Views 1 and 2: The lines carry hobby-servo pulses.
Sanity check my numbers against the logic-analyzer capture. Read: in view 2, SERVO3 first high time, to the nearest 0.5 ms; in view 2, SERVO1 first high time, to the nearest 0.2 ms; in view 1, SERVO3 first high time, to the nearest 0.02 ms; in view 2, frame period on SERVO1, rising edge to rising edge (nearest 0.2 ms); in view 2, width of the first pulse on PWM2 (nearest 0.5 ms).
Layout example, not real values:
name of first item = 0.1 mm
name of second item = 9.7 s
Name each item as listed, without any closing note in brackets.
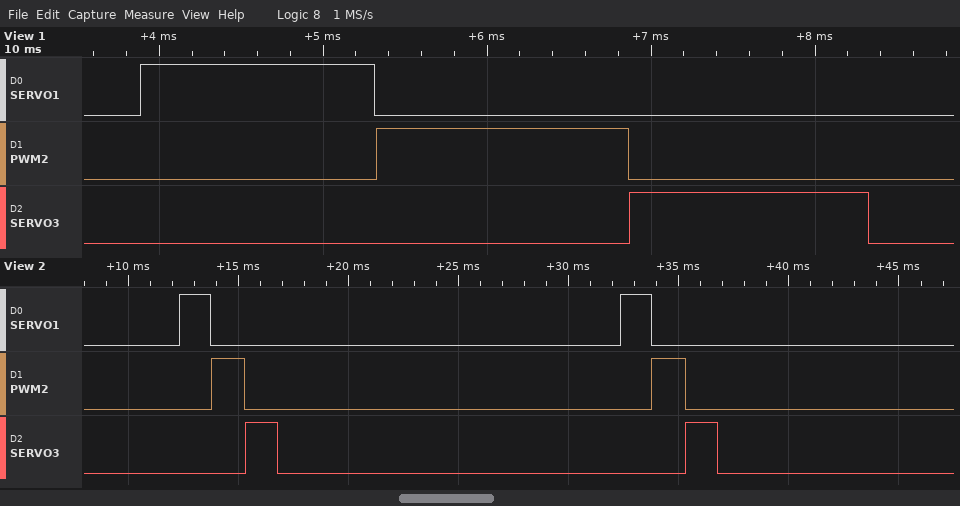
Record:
in view 2, SERVO3 first high time, to the nearest 0.5 ms = 1.5 ms
in view 2, SERVO1 first high time, to the nearest 0.2 ms = 1.4 ms
in view 1, SERVO3 first high time, to the nearest 0.02 ms = 1.46 ms
in view 2, frame period on SERVO1, rising edge to rising edge = 20.0 ms
in view 2, width of the first pulse on PWM2 = 1.5 ms
